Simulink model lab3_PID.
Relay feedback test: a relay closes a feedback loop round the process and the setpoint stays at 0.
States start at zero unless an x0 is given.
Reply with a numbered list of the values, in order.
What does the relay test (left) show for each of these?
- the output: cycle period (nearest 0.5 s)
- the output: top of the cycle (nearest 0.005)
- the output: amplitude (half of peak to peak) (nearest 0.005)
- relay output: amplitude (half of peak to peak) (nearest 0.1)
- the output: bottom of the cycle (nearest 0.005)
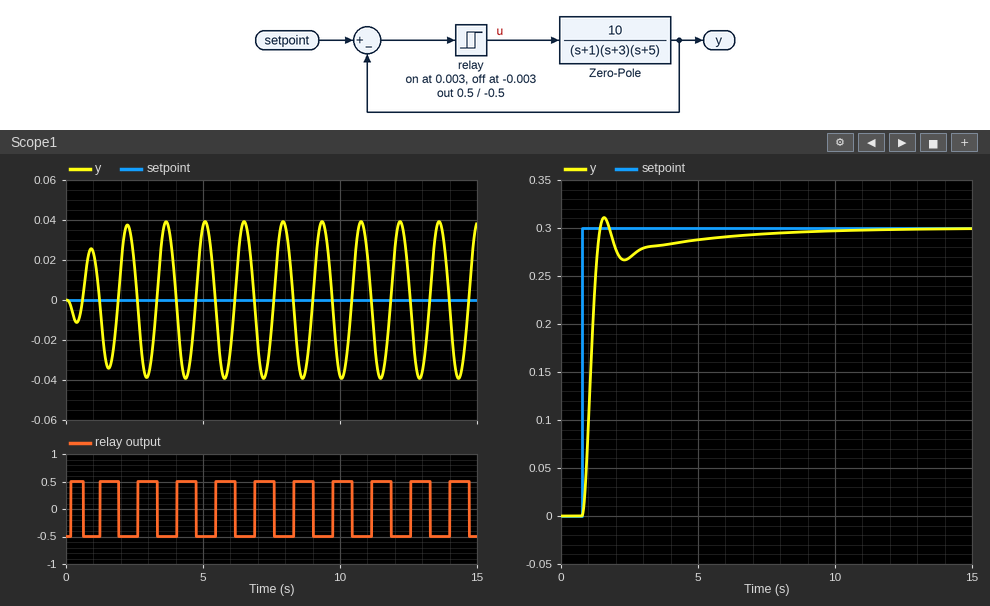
1. 1.5 s
2. 0.040
3. 0.040
4. 0.5
5. -0.040
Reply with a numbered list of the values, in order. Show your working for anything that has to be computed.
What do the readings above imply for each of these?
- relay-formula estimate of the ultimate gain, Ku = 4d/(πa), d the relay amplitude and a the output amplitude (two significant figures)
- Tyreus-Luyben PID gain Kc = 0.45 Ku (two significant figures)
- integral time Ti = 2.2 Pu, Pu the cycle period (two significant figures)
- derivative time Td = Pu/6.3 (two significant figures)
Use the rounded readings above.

1. 4 × 0.5 / (π × 0.04) = 16
2. 0.45 × 16 = 7.2
3. 2.2 × 1.5 = 3.3 s
4. 1.5 / 6.3 = 0.24 s
